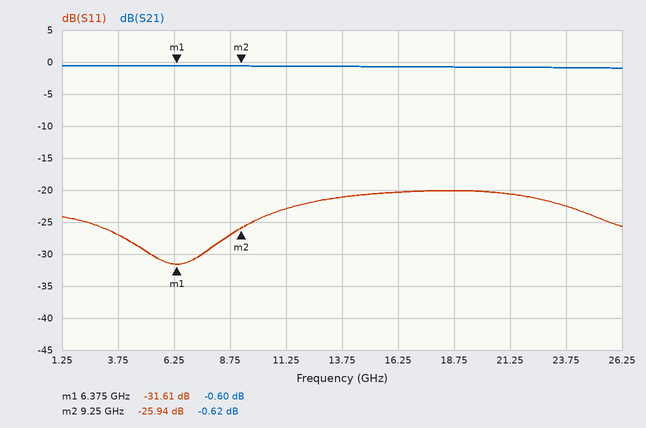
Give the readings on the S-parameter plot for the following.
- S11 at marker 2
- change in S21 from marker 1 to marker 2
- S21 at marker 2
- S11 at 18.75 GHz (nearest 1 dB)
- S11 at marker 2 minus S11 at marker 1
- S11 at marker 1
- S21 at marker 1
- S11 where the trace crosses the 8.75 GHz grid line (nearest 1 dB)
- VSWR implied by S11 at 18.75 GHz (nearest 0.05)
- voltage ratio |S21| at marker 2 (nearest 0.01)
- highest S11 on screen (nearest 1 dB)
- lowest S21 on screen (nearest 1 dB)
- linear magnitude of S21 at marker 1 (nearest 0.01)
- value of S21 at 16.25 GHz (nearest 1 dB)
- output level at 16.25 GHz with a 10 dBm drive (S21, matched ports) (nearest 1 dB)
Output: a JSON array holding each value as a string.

["-25.94 dB", "-0.02 dB", "-0.62 dB", "-20 dB", "5.67 dB", "-31.61 dB", "-0.60 dB", "-27 dB", "1.20", "0.93", "-20 dB", "-1 dB", "0.93", "-1 dB", "9 dBm"]
